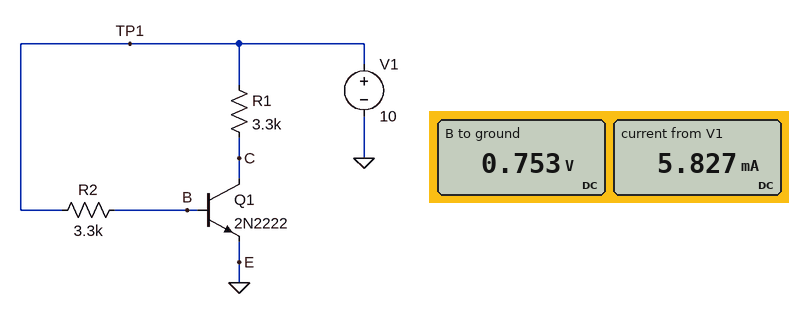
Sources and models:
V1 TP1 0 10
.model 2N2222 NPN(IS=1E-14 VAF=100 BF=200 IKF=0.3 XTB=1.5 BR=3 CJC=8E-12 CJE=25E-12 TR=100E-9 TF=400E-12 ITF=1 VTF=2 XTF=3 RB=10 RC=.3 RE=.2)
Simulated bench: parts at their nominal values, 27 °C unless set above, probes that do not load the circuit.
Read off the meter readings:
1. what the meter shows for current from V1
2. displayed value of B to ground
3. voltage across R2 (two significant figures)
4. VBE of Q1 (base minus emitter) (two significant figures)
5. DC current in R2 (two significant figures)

5.827 mA
0.753 V
9.2 V
750 mV
2.8 mA
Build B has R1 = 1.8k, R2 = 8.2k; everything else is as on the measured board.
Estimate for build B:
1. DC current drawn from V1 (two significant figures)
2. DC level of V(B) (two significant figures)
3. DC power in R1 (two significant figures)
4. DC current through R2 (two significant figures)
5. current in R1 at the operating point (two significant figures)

6.7 mA
730 mV
55 mW
1.1 mA
5.5 mA
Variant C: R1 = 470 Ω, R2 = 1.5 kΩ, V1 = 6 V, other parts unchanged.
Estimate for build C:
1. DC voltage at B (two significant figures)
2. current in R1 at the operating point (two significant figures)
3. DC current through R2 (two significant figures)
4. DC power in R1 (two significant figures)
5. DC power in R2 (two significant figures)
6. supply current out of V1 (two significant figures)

780 mV
13 mA
3.5 mA
76 mW
18 mW
16 mA
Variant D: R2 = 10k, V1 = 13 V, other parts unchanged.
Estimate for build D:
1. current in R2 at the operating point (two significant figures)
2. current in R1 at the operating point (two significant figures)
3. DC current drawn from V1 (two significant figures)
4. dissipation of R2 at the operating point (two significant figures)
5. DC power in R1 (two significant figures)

1.2 mA
3.9 mA
5.2 mA
15 mW
51 mW
